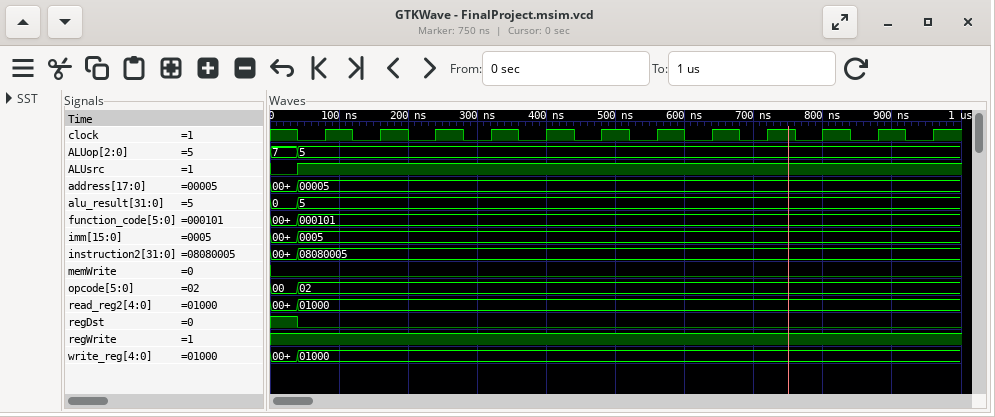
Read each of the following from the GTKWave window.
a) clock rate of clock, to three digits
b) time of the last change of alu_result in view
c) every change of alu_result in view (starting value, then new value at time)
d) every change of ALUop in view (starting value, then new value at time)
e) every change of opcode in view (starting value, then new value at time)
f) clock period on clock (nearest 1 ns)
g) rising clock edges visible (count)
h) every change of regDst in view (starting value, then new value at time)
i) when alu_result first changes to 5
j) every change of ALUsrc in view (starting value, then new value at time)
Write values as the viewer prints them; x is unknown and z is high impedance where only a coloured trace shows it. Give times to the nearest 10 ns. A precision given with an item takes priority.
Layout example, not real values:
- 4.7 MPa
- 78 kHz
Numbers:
- 12.5 MHz
- 40 ns
- 0, 5 at 40 ns
- 7, 5 at 40 ns
- 00, 02 at 40 ns
- 80 ns
- 12
- 1, 0 at 40 ns
- 40 ns
- 0, 1 at 40 ns
